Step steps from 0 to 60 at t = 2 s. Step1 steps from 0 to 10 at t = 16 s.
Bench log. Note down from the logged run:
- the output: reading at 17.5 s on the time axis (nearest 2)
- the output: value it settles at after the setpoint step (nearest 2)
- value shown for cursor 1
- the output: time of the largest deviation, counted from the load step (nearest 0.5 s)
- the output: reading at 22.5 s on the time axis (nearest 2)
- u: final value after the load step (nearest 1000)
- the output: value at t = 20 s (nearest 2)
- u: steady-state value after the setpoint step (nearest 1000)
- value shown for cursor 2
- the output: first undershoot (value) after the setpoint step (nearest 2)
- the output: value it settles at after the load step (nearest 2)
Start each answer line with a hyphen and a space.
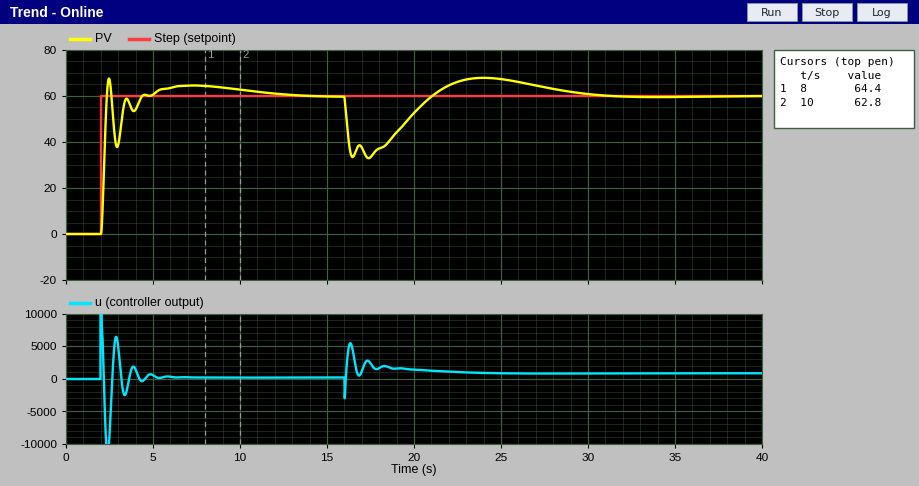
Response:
- 34
- 60
- 64.4
- 1.5 s
- 66
- 1000
- 52
- 0
- 62.8
- 38
- 60
